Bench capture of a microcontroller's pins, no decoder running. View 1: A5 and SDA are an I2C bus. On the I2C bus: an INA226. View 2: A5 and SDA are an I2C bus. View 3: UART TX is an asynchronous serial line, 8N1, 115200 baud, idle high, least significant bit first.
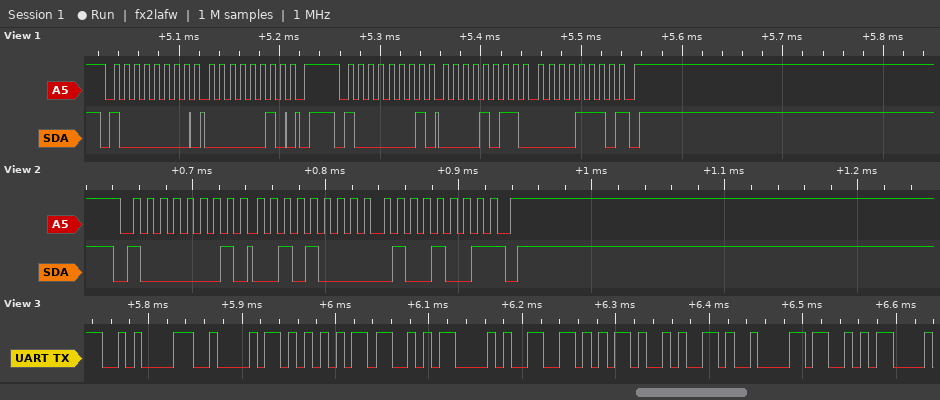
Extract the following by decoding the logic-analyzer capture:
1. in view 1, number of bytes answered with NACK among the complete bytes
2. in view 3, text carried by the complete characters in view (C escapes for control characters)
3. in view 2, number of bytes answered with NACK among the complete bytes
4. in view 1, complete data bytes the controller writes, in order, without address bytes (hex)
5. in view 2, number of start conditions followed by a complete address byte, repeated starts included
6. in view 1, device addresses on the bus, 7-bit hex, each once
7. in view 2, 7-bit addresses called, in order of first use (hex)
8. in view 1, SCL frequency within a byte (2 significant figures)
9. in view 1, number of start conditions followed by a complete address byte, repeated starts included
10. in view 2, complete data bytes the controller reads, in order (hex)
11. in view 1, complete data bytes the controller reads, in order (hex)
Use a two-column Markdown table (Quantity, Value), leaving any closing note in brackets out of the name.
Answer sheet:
| Quantity | Value |
|---|---|
| in view 1, number of bytes answered with NACK among the complete bytes | 1 |
| in view 3, text carried by the complete characters in view | "\nBUS(V)\tS" |
| in view 2, number of bytes answered with NACK among the complete bytes | 1 |
| in view 1, complete data bytes the controller writes, in order, without address bytes | 02 |
| in view 2, number of start conditions followed by a complete address byte, repeated starts included | 1 |
| in view 1, device addresses on the bus, 7-bit hex, each once | 0x40 |
| in view 2, 7-bit addresses called, in order of first use | 0x40 |
| in view 1, SCL frequency within a byte | 100 kHz |
| in view 1, number of start conditions followed by a complete address byte, repeated starts included | 2 |
| in view 2, complete data bytes the controller reads, in order | 28 49 |
| in view 1, complete data bytes the controller reads, in order | 0B 0E |
